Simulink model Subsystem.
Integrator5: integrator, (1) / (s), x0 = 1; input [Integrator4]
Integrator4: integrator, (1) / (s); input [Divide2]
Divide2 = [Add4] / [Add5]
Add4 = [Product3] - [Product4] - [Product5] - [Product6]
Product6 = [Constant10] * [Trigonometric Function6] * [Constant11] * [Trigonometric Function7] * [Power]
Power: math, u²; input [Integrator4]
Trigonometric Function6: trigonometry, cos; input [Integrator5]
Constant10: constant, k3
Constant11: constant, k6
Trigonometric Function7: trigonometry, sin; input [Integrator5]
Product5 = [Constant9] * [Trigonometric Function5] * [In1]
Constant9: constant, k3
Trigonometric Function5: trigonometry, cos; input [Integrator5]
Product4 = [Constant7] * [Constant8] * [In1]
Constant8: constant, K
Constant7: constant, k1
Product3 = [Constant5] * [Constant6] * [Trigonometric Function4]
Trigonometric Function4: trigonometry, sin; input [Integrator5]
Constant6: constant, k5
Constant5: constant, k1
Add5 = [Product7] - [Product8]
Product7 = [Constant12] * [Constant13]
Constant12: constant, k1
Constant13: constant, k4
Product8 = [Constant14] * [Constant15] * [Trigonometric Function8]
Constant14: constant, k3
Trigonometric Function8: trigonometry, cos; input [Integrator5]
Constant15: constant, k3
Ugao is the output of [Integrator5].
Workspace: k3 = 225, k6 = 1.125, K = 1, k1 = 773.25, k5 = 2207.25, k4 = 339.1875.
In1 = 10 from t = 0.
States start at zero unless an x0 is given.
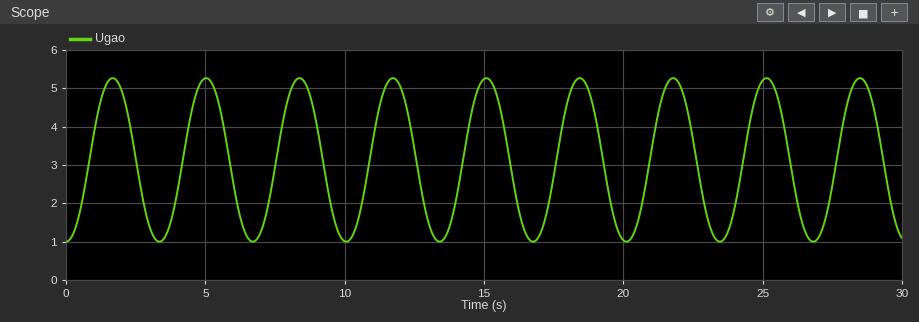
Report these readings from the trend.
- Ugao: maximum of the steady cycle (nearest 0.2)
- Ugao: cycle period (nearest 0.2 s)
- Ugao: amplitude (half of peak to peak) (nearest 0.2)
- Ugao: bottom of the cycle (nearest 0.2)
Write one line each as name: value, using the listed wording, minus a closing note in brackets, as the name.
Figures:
Ugao: maximum of the steady cycle: 5.2
Ugao: cycle period: 3.4 s
Ugao: amplitude (half of peak to peak): 2.2
Ugao: bottom of the cycle: 1.0
